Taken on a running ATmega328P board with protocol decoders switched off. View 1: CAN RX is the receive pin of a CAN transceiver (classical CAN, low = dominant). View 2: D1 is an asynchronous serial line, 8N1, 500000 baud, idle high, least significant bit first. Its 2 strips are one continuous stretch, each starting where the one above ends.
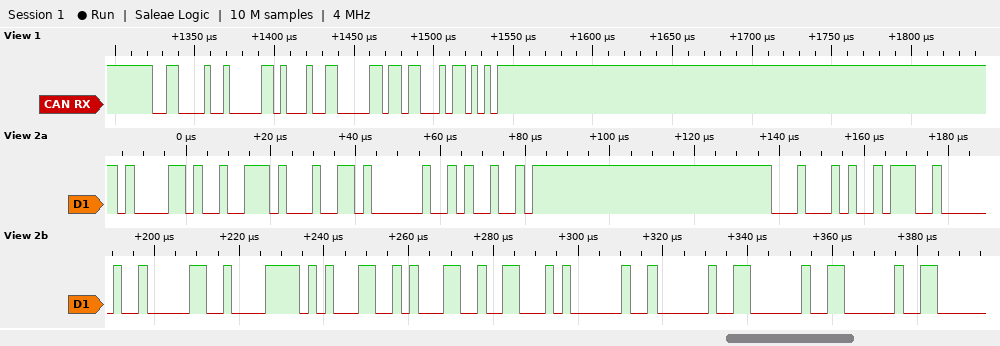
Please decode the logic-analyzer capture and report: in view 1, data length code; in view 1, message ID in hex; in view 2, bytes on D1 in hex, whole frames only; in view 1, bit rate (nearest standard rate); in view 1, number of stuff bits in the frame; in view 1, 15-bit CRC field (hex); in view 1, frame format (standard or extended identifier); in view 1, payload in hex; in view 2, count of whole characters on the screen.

2
0x309
61 72 64 20 49 44 3A 20 30 78 31 31 46 20 20 20 20
250 kbit/s
2
0x6C5A
standard
89 82
17
